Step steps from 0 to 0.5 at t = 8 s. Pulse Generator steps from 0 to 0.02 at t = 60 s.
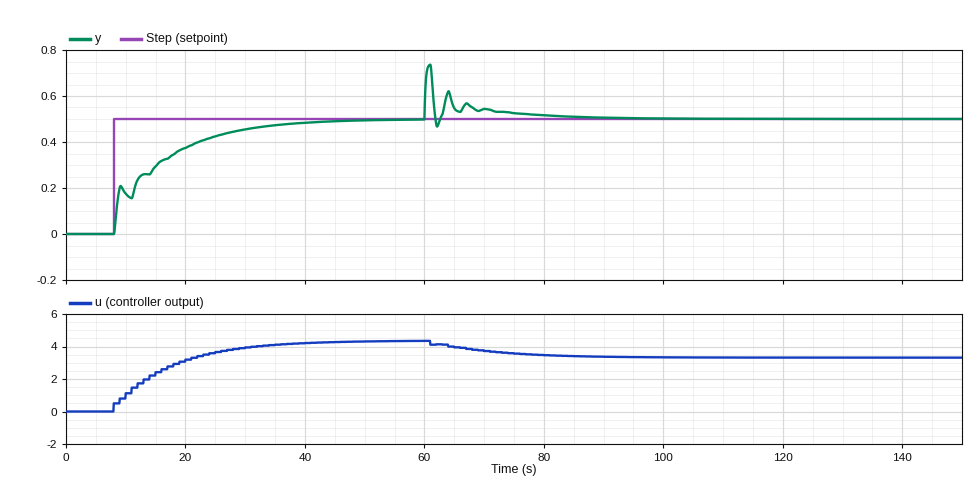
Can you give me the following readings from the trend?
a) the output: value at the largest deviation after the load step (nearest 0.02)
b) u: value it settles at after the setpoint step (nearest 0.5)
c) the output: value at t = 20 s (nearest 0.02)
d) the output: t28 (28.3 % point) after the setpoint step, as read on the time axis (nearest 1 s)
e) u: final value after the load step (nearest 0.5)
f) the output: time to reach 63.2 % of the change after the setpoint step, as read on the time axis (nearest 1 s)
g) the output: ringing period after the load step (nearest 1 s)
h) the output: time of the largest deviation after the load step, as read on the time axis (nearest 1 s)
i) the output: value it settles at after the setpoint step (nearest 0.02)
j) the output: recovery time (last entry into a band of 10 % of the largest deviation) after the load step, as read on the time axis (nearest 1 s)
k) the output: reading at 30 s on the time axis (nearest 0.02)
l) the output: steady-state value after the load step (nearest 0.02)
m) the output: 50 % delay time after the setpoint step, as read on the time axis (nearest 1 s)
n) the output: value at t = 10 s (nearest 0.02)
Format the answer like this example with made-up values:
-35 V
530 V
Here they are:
0.74
4.5
0.38
9 s
3.5
16 s
3 s
61 s
0.50
76 s
0.46
0.50
12 s
0.18
